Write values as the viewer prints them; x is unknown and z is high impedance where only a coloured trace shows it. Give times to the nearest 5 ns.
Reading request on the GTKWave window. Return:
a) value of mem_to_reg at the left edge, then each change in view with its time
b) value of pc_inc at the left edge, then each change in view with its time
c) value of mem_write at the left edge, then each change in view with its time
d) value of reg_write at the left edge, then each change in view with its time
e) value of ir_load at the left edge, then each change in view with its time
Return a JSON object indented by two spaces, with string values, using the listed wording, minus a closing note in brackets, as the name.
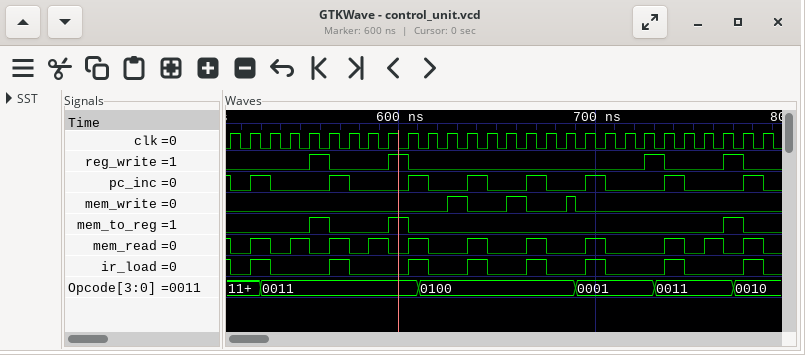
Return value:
{
  "value of mem_to_reg at the left edge, then each change in view with its time": "0, 1 at 555 ns, 0 at 565 ns, 1 at 595 ns, 0 at 605 ns, 1 at 765 ns, 0 at 775 ns",
  "value of pc_inc at the left edge, then each change in view with its time": "1, 0 at 515 ns, 1 at 525 ns, 0 at 535 ns, 1 at 565 ns, 0 at 575 ns, 1 at 605 ns, 0 at 615 ns, 1 at 635 ns, 0 at 645 ns, 1 at 665 ns, 0 at 675 ns, 1 at 695 ns, 0 at 705 ns, 1 at 735 ns, 0 at 745 ns, 1 at 775 ns, 0 at 785 ns",
  "value of mem_write at the left edge, then each change in view with its time": "0, 1 at 625 ns, 0 at 635 ns, 1 at 655 ns, 0 at 665 ns, 1 at 685 ns, 0 at 690 ns",
  "value of reg_write at the left edge, then each change in view with its time": "0, 1 at 555 ns, 0 at 565 ns, 1 at 595 ns, 0 at 605 ns, 1 at 725 ns, 0 at 735 ns, 1 at 765 ns, 0 at 775 ns",
  "value of ir_load at the left edge, then each change in view with its time": "1, 0 at 515 ns, 1 at 525 ns, 0 at 535 ns, 1 at 565 ns, 0 at 575 ns, 1 at 605 ns, 0 at 615 ns, 1 at 635 ns, 0 at 645 ns, 1 at 665 ns, 0 at 675 ns, 1 at 695 ns, 0 at 705 ns, 1 at 735 ns, 0 at 745 ns, 1 at 775 ns, 0 at 785 ns"
}
